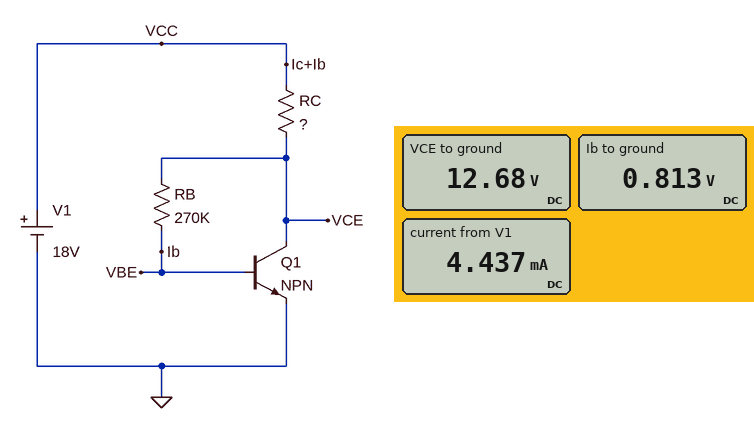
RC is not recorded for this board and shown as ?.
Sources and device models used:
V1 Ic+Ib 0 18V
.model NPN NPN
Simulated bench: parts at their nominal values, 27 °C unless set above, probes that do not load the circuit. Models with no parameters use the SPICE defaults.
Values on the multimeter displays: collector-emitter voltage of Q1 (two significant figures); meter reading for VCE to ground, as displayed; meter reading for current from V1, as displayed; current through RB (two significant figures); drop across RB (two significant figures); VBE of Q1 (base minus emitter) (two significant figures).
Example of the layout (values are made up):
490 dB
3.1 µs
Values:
13 V
12.68 V
4.437 mA
44 µA
12 V
810 mV
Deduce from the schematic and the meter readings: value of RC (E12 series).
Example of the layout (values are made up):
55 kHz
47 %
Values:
1.2 kΩ
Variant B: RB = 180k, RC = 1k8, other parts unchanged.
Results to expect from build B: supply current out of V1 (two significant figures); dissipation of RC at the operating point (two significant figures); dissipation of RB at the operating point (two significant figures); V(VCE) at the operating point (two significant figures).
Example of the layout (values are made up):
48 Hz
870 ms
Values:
4.8 mA
41 mW
410 µW
9.4 V
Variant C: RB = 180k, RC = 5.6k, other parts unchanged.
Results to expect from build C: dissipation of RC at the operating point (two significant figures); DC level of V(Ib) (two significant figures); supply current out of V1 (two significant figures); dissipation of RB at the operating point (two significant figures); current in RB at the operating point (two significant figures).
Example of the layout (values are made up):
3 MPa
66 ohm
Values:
30 mW
800 mV
2.3 mA
96 µW
23 µA
